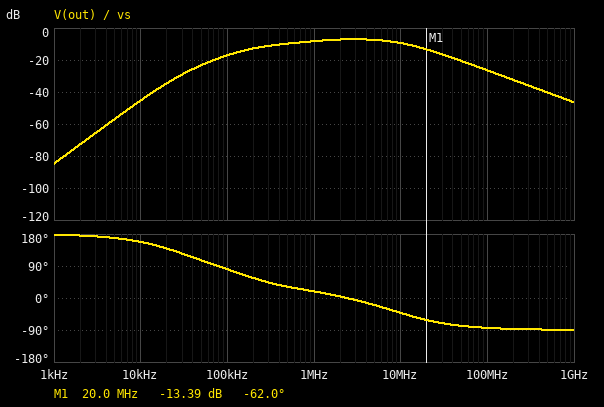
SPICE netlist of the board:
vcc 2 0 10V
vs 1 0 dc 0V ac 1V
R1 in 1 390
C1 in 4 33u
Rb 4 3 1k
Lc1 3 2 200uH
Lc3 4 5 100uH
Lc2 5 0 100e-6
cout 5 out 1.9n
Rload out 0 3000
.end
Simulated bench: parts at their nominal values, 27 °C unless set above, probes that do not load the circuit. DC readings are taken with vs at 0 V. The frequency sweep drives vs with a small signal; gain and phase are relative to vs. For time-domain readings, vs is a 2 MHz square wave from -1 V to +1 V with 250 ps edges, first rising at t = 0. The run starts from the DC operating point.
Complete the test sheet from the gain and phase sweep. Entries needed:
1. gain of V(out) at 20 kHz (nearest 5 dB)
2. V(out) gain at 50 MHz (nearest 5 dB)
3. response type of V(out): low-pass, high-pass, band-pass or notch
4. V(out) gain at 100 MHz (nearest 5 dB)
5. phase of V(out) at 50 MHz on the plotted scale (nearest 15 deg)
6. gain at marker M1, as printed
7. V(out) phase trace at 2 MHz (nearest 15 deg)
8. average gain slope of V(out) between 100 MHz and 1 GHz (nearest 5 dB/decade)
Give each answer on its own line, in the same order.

-35 dB
-20 dB
band-pass
-25 dB
-75 deg
-13.39 dB
0 deg
-20 dB/decade
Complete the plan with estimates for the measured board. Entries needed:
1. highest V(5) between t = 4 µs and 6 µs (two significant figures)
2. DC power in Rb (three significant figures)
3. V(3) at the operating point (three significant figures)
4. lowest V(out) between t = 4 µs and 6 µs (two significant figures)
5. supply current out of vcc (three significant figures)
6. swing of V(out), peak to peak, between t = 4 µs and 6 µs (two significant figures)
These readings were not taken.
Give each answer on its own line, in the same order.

540 mV
100 mW
10.0 V
-570 mV
10.0 mA
1.1 V
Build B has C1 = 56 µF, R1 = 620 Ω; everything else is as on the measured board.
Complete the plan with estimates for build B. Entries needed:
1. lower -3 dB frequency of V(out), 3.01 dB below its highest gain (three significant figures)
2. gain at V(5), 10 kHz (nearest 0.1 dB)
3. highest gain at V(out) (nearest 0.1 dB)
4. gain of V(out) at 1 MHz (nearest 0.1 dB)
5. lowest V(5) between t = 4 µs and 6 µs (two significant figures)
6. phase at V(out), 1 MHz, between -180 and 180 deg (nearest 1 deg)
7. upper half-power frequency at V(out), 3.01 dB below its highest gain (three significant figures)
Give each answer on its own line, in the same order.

766 kHz
-39.9 dB
-7.5 dB
-9.7 dB
-550 mV
27 deg
12.3 MHz
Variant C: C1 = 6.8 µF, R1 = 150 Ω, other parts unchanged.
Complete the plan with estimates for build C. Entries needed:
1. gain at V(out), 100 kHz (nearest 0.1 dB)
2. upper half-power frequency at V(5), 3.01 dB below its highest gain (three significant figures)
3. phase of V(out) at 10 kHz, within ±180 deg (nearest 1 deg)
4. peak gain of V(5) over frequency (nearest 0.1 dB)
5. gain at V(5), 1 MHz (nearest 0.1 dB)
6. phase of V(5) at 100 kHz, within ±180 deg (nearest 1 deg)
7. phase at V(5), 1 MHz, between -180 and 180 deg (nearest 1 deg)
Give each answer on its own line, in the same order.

-10.8 dB
10.5 MHz
156 deg
-6.5 dB
-6.8 dB
46 deg
4 deg
